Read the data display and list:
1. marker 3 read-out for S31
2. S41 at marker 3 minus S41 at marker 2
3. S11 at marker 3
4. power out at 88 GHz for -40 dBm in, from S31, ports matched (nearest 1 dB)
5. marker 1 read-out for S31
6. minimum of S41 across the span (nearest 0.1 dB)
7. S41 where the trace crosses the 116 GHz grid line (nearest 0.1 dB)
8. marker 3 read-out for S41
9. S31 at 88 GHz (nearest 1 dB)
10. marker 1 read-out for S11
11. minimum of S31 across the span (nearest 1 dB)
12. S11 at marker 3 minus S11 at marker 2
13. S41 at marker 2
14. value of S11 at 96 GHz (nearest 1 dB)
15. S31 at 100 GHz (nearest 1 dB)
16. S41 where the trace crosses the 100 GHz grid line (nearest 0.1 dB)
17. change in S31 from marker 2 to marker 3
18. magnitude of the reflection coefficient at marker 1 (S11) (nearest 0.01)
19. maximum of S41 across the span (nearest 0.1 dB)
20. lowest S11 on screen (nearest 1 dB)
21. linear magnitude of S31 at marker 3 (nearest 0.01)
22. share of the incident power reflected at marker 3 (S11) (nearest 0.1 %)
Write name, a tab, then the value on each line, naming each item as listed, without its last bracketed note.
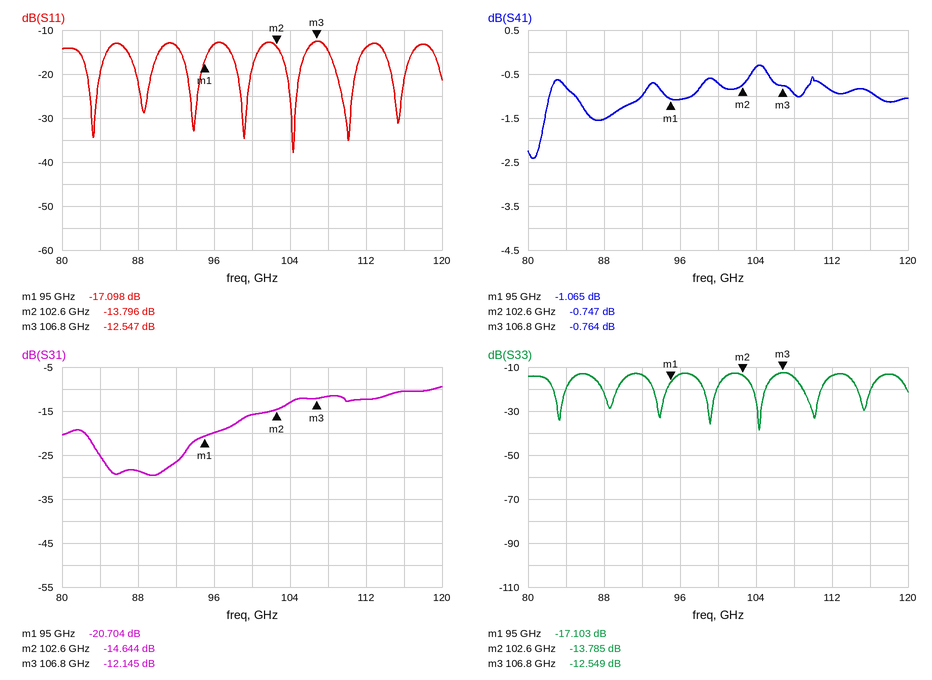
marker 3 read-out for S31	-12.145 dB
S41 at marker 3 minus S41 at marker 2	-0.017 dB
S11 at marker 3	-12.547 dB
power out at 88 GHz for -40 dBm in, from S31, ports matched	-69 dBm
marker 1 read-out for S31	-20.704 dB
minimum of S41 across the span	-2.4 dB
S41 where the trace crosses the 116 GHz grid line	-0.9 dB
marker 3 read-out for S41	-0.764 dB
S31 at 88 GHz	-29 dB
marker 1 read-out for S11	-17.098 dB
minimum of S31 across the span	-30 dB
S11 at marker 3 minus S11 at marker 2	1.249 dB
S41 at marker 2	-0.747 dB
value of S11 at 96 GHz	-13 dB
S31 at 100 GHz	-16 dB
S41 where the trace crosses the 100 GHz grid line	-0.7 dB
change in S31 from marker 2 to marker 3	2.499 dB
magnitude of the reflection coefficient at marker 1 (S11)	0.14
maximum of S41 across the span	-0.3 dB
lowest S11 on screen	-38 dB
linear magnitude of S31 at marker 3	0.25
share of the incident power reflected at marker 3 (S11)	5.6 %
